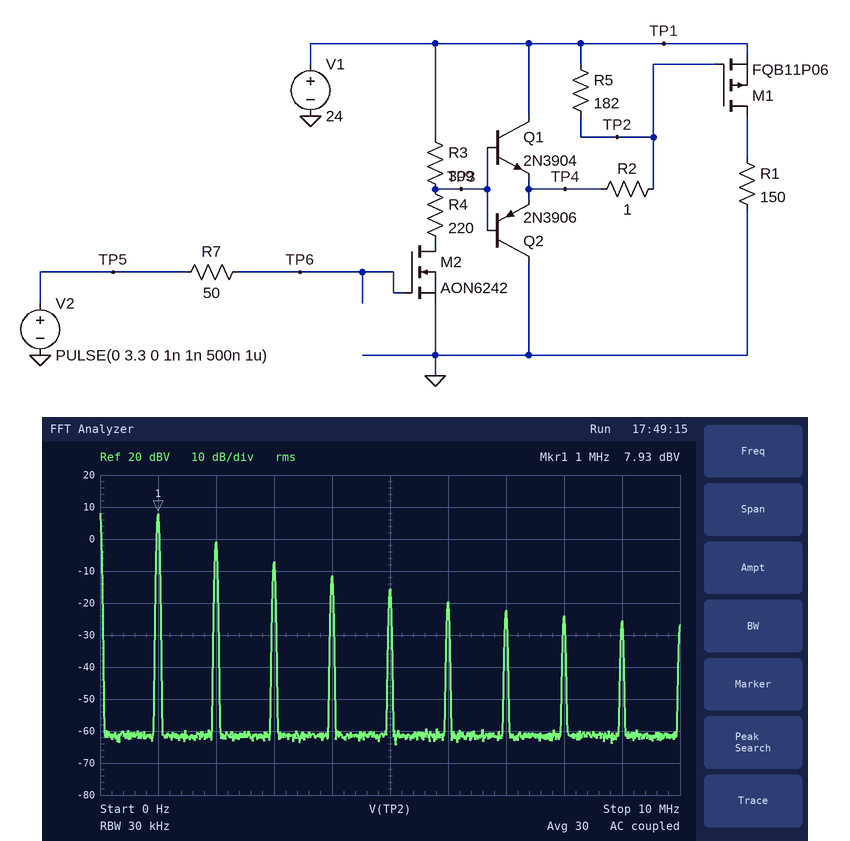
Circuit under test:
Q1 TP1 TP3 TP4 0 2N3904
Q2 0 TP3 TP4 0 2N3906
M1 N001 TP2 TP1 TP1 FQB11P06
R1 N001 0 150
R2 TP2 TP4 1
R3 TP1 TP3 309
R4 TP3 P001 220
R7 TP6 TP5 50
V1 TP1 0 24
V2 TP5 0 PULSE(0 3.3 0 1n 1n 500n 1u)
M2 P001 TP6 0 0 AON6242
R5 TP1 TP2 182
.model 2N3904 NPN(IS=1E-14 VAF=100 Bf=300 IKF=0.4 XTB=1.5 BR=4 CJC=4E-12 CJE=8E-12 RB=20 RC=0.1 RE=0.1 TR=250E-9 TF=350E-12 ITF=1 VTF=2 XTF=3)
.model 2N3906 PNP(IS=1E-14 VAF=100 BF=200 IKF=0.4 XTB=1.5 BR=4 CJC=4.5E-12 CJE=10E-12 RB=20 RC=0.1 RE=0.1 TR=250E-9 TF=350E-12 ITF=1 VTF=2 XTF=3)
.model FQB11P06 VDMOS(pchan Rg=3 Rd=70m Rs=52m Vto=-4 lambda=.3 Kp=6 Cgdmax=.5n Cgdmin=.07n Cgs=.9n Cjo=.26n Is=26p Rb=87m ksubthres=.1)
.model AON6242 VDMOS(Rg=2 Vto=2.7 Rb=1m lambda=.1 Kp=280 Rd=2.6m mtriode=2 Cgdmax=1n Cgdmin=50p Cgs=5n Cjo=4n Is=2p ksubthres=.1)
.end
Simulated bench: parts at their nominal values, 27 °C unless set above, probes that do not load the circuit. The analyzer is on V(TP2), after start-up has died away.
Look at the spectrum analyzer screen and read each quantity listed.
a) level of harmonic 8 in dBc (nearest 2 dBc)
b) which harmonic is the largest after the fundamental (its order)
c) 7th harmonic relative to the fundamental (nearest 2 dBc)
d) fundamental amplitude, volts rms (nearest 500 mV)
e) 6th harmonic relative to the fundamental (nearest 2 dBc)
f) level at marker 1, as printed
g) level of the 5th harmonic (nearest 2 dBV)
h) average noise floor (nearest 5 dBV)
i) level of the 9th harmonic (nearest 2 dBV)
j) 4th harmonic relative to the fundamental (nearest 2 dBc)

-32 dBc
2
-30 dBc
2.5 V
-28 dBc
7.93 dBV
-16 dBV
-60 dBV
-26 dBV
-20 dBc
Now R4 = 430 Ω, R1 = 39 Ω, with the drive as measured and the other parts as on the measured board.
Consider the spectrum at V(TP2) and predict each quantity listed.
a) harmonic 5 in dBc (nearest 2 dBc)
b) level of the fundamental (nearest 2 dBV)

-22 dBc
2 dBV
